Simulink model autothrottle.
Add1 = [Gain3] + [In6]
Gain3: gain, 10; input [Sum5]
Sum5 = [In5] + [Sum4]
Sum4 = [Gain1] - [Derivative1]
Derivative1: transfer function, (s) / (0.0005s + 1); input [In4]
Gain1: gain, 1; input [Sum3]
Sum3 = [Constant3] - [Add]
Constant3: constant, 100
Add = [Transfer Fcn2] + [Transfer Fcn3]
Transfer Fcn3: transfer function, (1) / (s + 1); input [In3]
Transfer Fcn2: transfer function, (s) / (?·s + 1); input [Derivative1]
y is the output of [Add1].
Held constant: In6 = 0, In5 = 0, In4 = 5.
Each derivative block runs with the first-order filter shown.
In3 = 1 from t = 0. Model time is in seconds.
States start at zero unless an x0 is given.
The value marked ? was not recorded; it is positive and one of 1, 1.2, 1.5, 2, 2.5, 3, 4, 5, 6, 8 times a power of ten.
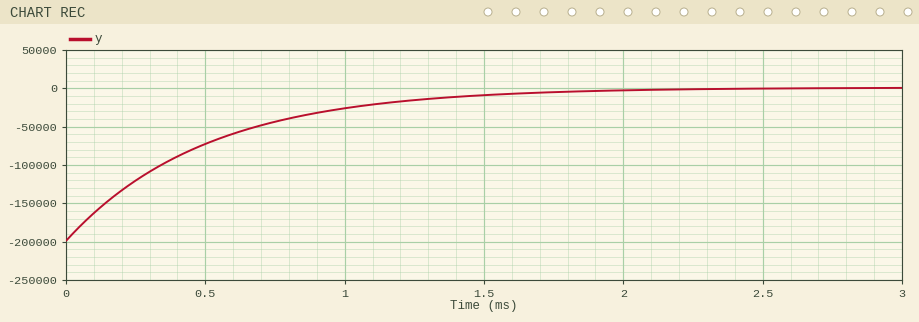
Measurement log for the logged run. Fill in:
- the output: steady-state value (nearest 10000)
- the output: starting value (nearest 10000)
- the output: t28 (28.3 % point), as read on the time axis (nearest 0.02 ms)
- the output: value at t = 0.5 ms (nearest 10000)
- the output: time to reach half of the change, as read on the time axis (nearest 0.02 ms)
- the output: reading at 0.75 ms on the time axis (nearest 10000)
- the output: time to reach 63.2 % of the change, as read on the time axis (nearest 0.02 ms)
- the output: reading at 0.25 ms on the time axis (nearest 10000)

0
-200000
0.16 ms
-70000
0.34 ms
-40000
0.50 ms
-120000
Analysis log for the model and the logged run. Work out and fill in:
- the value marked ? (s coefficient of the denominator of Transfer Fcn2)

1
